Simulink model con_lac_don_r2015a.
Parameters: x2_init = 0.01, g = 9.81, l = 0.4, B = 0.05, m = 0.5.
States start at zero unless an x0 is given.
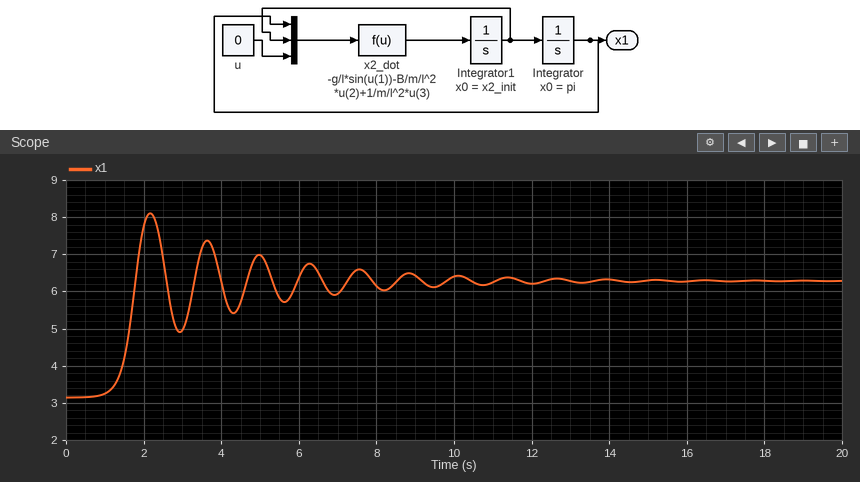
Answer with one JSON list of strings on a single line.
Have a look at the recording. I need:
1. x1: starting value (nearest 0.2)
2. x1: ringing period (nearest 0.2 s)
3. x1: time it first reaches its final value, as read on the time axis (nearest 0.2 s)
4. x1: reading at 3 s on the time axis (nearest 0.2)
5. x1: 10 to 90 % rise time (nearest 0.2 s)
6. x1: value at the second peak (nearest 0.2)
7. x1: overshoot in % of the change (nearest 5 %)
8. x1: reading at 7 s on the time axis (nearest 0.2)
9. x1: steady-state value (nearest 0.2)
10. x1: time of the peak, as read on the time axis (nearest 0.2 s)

["3.2", "1.4 s", "1.8 s", "5.0", "0.6 s", "7.4", "60 %", "6.0", "6.2", "2.2 s"]
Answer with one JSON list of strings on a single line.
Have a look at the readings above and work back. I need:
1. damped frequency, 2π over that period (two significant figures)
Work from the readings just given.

["4.5 rad/s"]
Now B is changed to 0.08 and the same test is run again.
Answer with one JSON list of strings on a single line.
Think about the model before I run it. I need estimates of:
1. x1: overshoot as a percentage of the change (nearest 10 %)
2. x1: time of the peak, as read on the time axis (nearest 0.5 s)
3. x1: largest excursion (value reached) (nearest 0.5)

["50 %", "2.0 s", "8.0"]
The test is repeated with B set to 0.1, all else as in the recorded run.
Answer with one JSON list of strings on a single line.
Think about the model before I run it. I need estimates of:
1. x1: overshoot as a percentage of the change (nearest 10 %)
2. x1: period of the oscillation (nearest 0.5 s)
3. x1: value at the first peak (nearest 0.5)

["40 %", "1.5 s", "7.5"]
